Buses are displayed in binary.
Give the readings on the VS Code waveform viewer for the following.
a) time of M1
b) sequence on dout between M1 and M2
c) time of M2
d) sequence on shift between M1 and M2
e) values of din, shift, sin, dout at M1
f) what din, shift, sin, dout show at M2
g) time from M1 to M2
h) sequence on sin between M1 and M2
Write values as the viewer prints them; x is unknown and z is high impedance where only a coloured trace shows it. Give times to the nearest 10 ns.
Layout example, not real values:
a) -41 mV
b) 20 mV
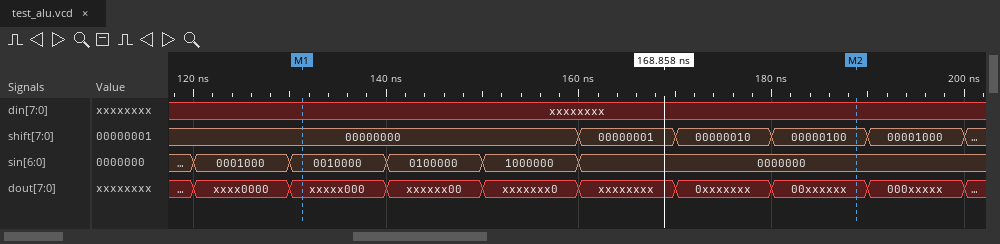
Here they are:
a) 130 ns
b) xxxxx000, xxxxxx00, xxxxxxx0, xxxxxxxx, 0xxxxxxx, 00xxxxxx
c) 190 ns
d) 00000000, 00000001, 00000010, 00000100
e) din=xxxxxxxx, shift=00000000, sin=0010000, dout=xxxxx000
f) din=xxxxxxxx, shift=00000100, sin=0000000, dout=00xxxxxx
g) 60 ns
h) 0010000, 0100000, 1000000, 0000000
